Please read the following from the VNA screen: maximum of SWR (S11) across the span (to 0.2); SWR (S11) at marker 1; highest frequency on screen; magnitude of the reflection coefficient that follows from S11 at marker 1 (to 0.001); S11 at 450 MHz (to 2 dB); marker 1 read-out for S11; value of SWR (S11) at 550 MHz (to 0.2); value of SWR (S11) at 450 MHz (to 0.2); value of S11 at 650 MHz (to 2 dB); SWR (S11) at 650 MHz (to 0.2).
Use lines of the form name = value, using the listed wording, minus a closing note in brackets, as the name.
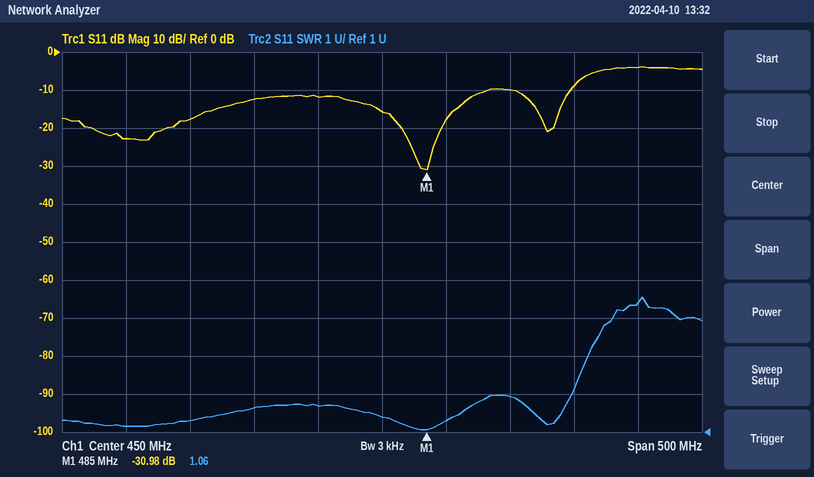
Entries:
maximum of SWR (S11) across the span = 4.6
SWR (S11) at marker 1 = 1.06
highest frequency on screen = 700 MHz
magnitude of the reflection coefficient that follows from S11 at marker 1 = 0.028
S11 at 450 MHz = -16 dB
marker 1 read-out for S11 = -30.98 dB
value of SWR (S11) at 550 MHz = 2.0
value of SWR (S11) at 450 MHz = 1.4
value of S11 at 650 MHz = -4 dB
SWR (S11) at 650 MHz = 4.4
